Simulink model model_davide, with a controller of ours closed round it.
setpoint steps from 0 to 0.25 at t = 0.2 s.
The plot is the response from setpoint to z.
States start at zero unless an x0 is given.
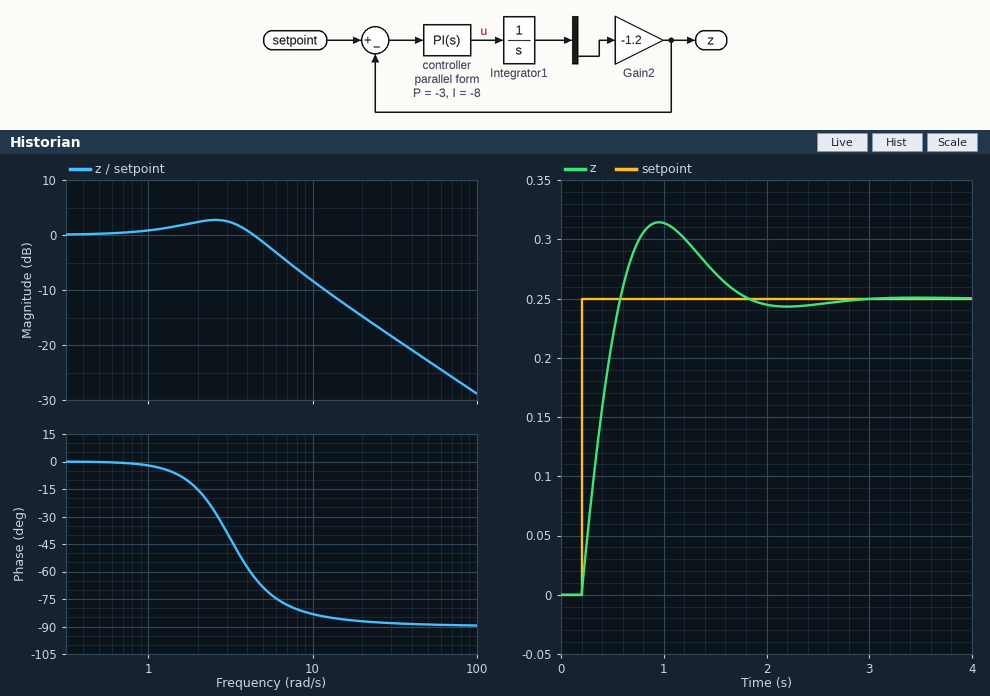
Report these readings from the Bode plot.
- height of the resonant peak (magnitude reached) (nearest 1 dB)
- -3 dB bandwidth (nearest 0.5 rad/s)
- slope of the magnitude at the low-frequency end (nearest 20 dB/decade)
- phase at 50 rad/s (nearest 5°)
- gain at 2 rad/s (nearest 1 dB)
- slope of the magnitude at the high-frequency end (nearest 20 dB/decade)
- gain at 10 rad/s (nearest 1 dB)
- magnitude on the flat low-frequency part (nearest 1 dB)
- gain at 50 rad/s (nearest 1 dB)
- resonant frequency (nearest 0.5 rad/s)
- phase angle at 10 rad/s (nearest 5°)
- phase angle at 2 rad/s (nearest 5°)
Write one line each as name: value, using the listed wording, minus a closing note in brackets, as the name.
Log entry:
height of the resonant peak (magnitude reached): 3 dB
-3 dB bandwidth: 6.0 rad/s
slope of the magnitude at the low-frequency end: 0 dB/decade
phase at 50 rad/s: -90°
gain at 2 rad/s: 2 dB
slope of the magnitude at the high-frequency end: -20 dB/decade
gain at 10 rad/s: -8 dB
magnitude on the flat low-frequency part: 0 dB
gain at 50 rad/s: -23 dB
resonant frequency: 2.5 rad/s
phase angle at 10 rad/s: -85°
phase angle at 2 rad/s: -15°
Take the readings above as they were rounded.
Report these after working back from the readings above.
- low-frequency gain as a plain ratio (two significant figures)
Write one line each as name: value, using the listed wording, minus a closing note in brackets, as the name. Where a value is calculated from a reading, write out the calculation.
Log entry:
low-frequency gain as a plain ratio: 10^(0 / 20) = 1.0
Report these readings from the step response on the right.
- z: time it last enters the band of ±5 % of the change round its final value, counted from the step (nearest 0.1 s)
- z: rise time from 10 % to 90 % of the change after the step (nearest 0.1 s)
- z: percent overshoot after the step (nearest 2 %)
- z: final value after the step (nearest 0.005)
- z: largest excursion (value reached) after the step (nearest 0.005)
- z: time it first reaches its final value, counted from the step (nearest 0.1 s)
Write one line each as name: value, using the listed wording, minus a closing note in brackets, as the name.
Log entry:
z: time it last enters the band of ±5 % of the change round its final value, counted from the step: 1.4 s
z: rise time from 10 % to 90 % of the change after the step: 0.3 s
z: percent overshoot after the step: 26 %
z: final value after the step: 0.250
z: largest excursion (value reached) after the step: 0.315
z: time it first reaches its final value, counted from the step: 0.4 s
